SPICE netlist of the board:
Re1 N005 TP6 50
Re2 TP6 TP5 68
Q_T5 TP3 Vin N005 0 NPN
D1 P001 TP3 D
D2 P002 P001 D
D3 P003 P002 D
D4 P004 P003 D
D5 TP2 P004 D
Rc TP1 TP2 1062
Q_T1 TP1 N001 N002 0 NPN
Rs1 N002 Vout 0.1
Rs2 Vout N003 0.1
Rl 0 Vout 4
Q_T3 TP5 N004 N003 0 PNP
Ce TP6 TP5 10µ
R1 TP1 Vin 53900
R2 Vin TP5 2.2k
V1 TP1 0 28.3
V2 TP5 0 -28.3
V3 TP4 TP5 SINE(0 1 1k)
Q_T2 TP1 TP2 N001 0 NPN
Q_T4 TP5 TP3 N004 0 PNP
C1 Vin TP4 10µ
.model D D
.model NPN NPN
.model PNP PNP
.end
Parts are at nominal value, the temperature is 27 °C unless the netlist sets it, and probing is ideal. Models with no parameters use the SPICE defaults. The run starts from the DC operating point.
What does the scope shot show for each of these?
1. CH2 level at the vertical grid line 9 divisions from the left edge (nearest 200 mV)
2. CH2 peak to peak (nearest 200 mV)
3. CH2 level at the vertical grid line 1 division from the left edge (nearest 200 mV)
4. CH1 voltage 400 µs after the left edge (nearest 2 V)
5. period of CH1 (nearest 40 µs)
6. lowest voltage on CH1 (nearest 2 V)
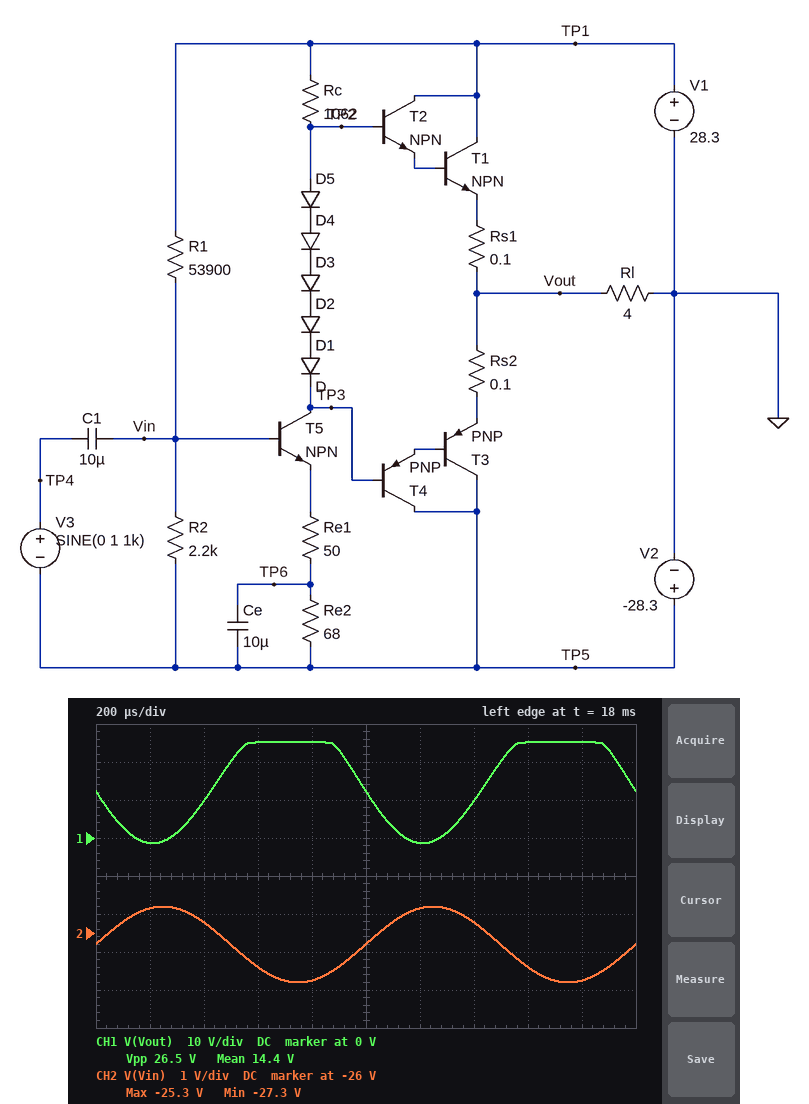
-27.2 V
2.0 V
-25.4 V
10 V
1.00 ms
-2 V
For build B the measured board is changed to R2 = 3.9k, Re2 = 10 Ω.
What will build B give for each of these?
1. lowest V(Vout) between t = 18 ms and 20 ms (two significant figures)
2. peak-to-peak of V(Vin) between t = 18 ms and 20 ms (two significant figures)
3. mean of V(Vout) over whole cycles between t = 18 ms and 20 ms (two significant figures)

-23 V
2.0 V
-5.6 V
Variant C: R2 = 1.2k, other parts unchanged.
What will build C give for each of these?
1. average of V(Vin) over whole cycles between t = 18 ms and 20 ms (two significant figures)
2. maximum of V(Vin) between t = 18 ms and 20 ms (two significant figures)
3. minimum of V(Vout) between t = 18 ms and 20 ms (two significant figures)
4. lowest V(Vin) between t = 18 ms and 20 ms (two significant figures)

-27 V
-26 V
7.4 V
-28 V
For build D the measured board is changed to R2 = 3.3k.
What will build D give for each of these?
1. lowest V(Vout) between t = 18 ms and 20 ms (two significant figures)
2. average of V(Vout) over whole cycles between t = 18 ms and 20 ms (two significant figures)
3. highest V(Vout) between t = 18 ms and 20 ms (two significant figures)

-8.6 V
8.8 V
25 V
